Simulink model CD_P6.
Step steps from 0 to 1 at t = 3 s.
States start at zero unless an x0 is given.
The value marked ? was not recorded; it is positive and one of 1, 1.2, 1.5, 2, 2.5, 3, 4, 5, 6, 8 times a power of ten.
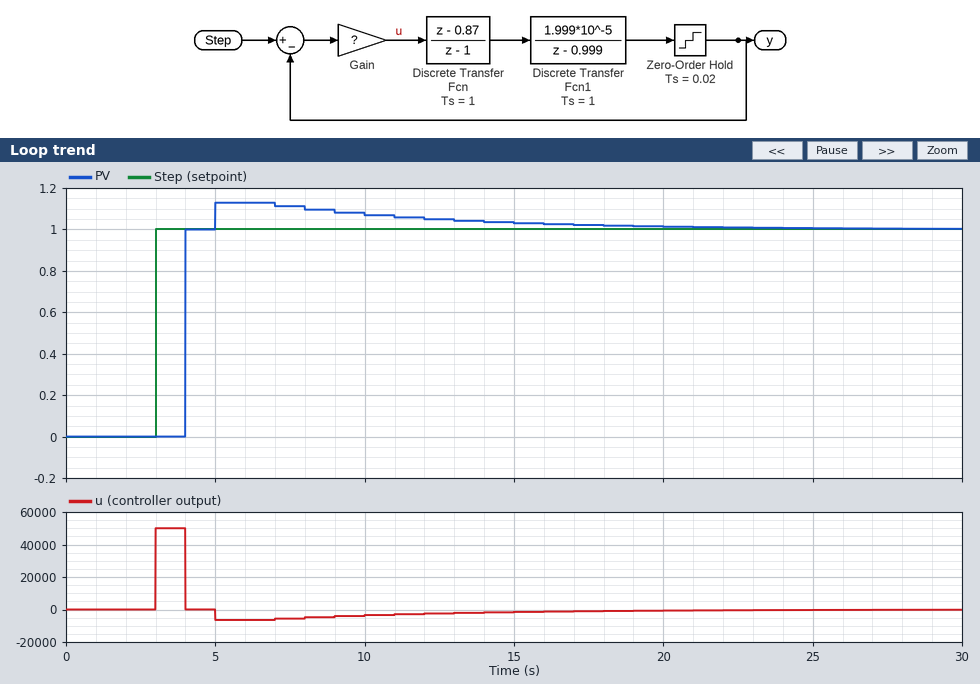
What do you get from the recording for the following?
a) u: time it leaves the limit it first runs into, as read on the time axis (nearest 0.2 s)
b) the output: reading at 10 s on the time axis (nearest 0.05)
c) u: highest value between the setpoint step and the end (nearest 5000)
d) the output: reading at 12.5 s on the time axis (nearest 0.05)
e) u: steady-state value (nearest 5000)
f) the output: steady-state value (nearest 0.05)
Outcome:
4.0 s
1.05
50000
1.05
0
1.00
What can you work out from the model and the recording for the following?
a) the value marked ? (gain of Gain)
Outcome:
50000
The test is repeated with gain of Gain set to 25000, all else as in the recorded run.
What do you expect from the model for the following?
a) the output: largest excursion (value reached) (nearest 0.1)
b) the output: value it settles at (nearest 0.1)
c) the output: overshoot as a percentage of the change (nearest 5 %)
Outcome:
1.2
1.0
20 %
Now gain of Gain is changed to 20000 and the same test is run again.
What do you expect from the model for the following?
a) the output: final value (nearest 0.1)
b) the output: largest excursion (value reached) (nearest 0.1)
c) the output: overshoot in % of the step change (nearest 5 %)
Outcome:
1.0
1.2
20 %
